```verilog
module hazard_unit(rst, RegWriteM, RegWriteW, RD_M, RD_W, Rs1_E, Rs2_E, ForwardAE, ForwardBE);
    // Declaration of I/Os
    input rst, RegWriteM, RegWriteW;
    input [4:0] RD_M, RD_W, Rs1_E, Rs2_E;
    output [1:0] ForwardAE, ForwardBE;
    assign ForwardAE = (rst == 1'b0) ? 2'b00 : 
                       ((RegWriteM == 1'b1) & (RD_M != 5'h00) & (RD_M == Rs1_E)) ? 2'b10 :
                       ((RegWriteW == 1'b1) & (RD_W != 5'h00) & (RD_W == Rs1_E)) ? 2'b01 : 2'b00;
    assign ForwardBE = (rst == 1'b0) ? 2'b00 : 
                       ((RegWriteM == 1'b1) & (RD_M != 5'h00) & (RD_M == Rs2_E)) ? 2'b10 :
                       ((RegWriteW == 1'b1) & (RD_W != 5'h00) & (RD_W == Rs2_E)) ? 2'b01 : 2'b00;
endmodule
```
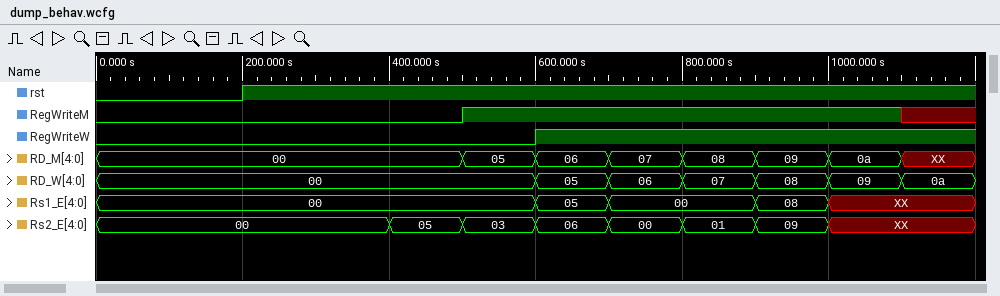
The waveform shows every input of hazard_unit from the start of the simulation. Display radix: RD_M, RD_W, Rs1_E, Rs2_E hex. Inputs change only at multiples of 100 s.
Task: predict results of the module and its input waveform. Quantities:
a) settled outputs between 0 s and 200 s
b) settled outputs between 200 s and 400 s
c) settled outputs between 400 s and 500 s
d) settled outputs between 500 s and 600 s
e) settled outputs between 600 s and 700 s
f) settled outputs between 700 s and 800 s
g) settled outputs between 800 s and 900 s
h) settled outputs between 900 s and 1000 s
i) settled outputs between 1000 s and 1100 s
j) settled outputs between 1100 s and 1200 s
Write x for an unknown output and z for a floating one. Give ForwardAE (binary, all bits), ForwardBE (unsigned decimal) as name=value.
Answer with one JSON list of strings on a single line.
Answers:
["ForwardAE=00, ForwardBE=0", "ForwardAE=00, ForwardBE=0", "ForwardAE=00, ForwardBE=0", "ForwardAE=00, ForwardBE=0", "ForwardAE=01, ForwardBE=2", "ForwardAE=00, ForwardBE=0", "ForwardAE=00, ForwardBE=0", "ForwardAE=01, ForwardBE=2", "ForwardAE=x, ForwardBE=x", "ForwardAE=x, ForwardBE=x"]
